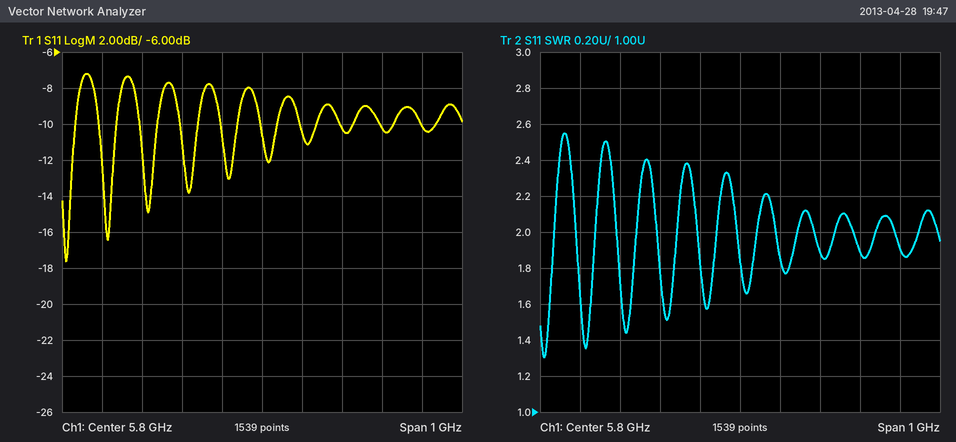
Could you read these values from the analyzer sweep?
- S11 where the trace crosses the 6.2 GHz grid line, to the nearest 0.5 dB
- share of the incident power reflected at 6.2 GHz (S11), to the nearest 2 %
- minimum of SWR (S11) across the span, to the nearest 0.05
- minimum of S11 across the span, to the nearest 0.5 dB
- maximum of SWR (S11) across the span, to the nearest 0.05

-10.0 dB
10 %
1.30
-17.5 dB
2.55
